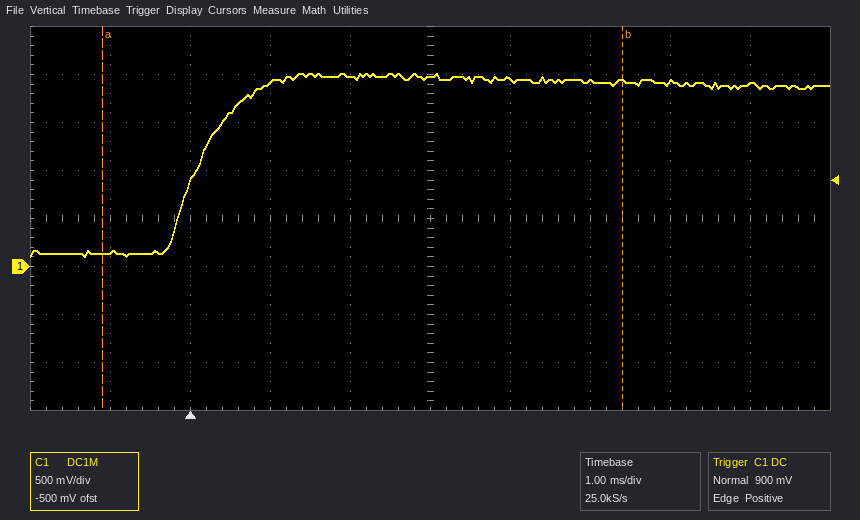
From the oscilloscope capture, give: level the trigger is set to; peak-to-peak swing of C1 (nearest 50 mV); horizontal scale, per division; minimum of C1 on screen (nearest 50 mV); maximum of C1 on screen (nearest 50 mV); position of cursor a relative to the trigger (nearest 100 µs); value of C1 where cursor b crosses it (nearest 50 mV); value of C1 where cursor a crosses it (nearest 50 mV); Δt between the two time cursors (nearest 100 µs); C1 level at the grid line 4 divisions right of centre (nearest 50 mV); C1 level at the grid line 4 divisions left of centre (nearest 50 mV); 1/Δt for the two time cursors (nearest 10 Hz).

900 mV
1.90 V
1 ms
100 mV
2.00 V
-1.1 ms
1.95 V
150 mV
6.5 ms
1.90 V
150 mV
150 Hz
